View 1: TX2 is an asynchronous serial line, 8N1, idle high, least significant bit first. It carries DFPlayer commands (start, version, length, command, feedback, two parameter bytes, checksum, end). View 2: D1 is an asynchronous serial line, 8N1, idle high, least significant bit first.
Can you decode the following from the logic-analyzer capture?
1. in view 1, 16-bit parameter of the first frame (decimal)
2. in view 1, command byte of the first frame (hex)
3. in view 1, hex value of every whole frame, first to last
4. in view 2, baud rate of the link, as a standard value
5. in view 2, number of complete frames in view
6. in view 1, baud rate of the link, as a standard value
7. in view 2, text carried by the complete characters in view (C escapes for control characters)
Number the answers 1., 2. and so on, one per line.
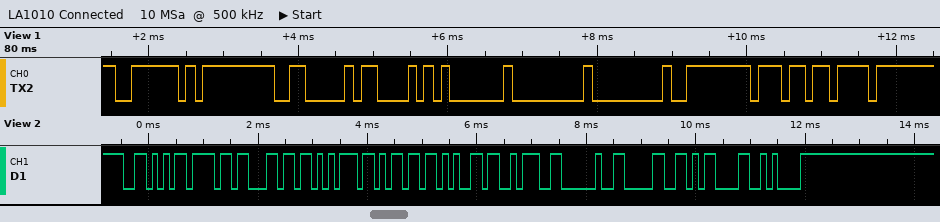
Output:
1. 0
2. 0x43
3. 7E FF 06 43 01 00 00 FE B7 EF
4. 9600 baud
5. 11
6. 9600 baud
7. "Volume: 0\r\n"
